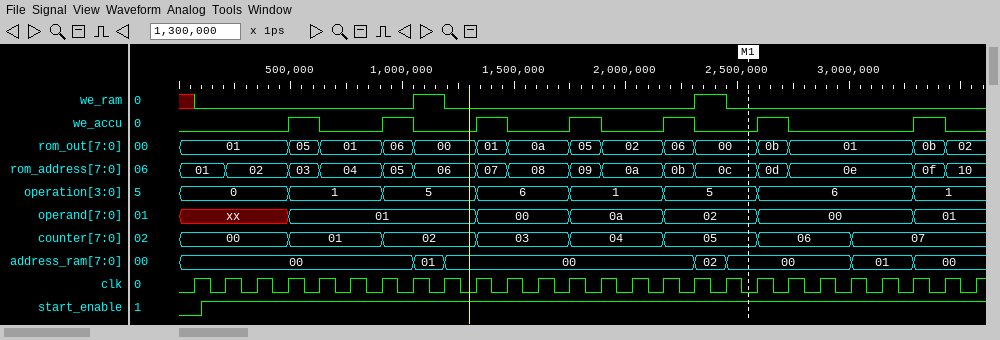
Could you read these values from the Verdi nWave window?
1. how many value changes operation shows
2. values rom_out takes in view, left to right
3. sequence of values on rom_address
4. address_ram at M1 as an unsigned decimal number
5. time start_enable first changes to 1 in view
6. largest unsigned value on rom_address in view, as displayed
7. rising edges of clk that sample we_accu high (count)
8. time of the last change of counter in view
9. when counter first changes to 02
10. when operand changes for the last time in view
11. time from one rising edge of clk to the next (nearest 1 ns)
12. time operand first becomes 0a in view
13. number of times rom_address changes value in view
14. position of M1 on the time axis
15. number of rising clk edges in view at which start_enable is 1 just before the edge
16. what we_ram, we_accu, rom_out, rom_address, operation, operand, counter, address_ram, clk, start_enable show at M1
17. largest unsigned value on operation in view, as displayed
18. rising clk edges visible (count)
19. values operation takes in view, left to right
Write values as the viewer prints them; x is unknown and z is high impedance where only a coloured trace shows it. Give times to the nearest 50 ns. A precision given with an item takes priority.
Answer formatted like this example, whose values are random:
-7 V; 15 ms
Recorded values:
7; 01, 05, 01, 06, 00, 01, 0a, 05, 02, 06, 00, 0b, 01, 0b, 02; 01, 02, 03, 04, 05, 06, 07, 08, 09, 0a, 0b, 0c, 0d, 0e, 0f, 10; 0; 100 ns; 10; 7; 3000 ns; 900 ns; 3300 ns; 140 ns; 1750 ns; 15; 2550 ns; 25; we_ram=0, we_accu=0, rom_out=00, rom_address=0c, operation=5, operand=02, counter=05, address_ram=00, clk=0, start_enable=1; 6; 26; 0, 1, 5, 6, 1, 5, 6, 1
